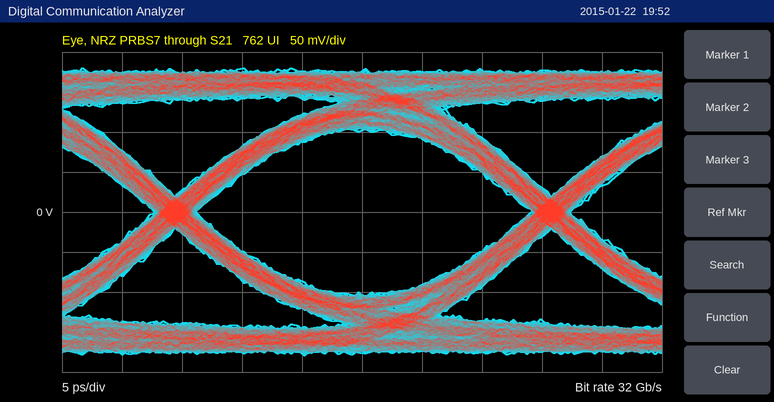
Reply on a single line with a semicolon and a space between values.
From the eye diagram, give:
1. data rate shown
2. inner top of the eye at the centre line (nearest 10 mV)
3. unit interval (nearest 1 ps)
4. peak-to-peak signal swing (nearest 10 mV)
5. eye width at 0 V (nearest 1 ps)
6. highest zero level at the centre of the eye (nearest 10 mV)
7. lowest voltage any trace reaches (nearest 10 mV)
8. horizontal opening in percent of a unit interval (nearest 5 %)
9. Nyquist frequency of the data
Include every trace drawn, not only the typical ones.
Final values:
32 Gb/s; 100 mV; 31 ps; 360 mV; 28 ps; -100 mV; -180 mV; 90 %; 16 GHz
